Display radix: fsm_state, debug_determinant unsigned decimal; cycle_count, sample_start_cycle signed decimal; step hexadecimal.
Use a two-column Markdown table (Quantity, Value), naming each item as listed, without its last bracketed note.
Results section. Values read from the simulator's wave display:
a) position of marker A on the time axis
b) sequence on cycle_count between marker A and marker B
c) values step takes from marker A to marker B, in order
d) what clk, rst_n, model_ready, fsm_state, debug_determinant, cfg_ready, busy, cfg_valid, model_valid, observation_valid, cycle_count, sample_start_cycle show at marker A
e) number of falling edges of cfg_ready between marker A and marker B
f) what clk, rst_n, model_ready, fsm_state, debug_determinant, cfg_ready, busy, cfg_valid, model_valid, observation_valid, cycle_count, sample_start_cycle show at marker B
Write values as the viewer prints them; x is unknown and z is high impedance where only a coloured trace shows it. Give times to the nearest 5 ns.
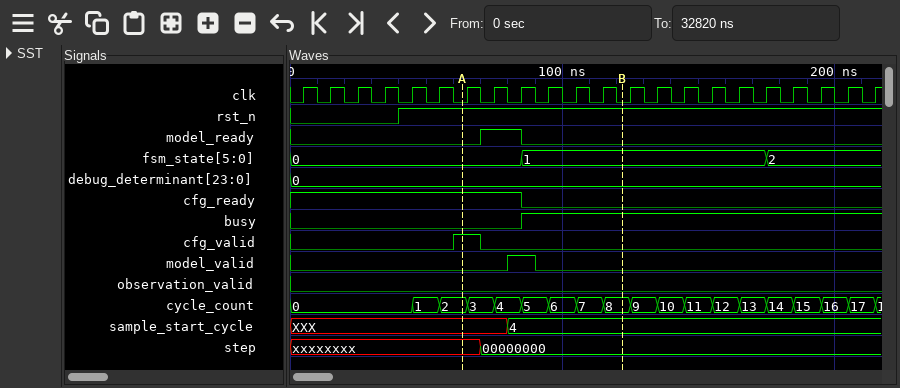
| Quantity | Value |
|---|---|
| position of marker A on the time axis | 65 ns |
| sequence on cycle_count between marker A and marker B | 2, 3, 4, 5, 6, 7, 8 |
| values step takes from marker A to marker B, in order | xxxxxxxx, 00000000 |
| what clk, rst_n, model_ready, fsm_state, debug_determinant, cfg_ready, busy, cfg_valid, model_valid, observation_valid, cycle_count, sample_start_cycle show at marker A | clk=0, rst_n=1, model_ready=0, fsm_state=0, debug_determinant=0, cfg_ready=1, busy=0, cfg_valid=1, model_valid=0, observation_valid=0, cycle_count=2, sample_start_cycle=XXX |
| number of falling edges of cfg_ready between marker A and marker B | 1 |
| what clk, rst_n, model_ready, fsm_state, debug_determinant, cfg_ready, busy, cfg_valid, model_valid, observation_valid, cycle_count, sample_start_cycle show at marker B | clk=0, rst_n=1, model_ready=0, fsm_state=1, debug_determinant=0, cfg_ready=0, busy=1, cfg_valid=0, model_valid=0, observation_valid=0, cycle_count=8, sample_start_cycle=4 |
